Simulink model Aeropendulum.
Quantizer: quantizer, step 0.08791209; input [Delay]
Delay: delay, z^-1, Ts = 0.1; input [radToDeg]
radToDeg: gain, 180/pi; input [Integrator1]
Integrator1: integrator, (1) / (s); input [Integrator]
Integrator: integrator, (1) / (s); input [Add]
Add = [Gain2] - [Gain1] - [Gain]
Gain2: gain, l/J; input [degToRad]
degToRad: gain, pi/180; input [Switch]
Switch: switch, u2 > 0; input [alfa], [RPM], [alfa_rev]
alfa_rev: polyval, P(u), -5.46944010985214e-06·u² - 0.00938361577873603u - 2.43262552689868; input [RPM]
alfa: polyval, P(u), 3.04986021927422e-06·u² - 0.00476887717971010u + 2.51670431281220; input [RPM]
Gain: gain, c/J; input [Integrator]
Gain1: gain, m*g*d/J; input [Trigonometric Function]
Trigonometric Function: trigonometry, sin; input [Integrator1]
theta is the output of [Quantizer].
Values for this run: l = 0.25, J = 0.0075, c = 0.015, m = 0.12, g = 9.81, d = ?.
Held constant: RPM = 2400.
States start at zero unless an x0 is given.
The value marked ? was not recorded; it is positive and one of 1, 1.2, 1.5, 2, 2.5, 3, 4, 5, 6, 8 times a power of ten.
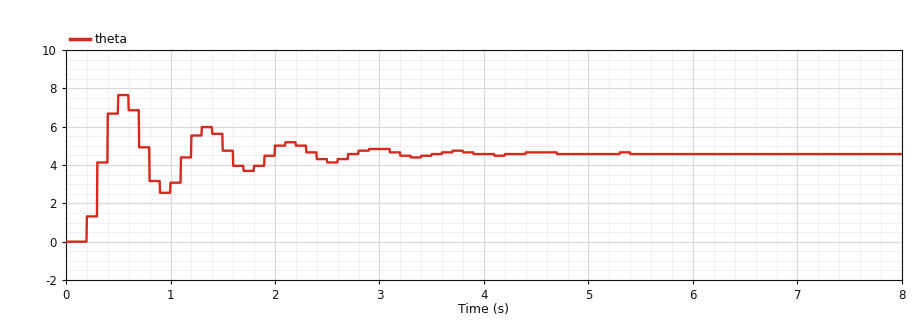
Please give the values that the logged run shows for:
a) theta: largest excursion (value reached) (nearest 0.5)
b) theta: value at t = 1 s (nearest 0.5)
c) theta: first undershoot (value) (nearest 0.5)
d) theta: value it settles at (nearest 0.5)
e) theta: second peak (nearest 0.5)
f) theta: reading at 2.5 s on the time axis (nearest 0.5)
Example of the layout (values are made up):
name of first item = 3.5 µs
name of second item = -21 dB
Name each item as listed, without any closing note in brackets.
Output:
theta: largest excursion (value reached) = 7.5
theta: value at t = 1 s = 3.0
theta: first undershoot (value) = 2.5
theta: value it settles at = 4.5
theta: second peak = 6.0
theta: reading at 2.5 s on the time axis = 4.0
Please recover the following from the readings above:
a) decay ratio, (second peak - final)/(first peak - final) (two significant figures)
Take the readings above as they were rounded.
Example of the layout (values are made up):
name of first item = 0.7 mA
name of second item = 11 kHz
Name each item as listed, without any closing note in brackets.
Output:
decay ratio, (second peak - final)/(first peak - final) = 0.50
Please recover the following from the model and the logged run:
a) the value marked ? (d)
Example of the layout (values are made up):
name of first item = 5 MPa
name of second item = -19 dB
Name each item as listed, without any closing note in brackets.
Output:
the value marked ? = 0.4
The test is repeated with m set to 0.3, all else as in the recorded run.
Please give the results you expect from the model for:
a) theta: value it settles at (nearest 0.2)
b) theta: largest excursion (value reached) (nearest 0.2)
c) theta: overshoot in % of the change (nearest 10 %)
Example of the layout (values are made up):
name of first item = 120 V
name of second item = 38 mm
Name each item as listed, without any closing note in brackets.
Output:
theta: value it settles at = 1.8
theta: largest excursion (value reached) = 3.0
theta: overshoot in % of the change = 60 %
